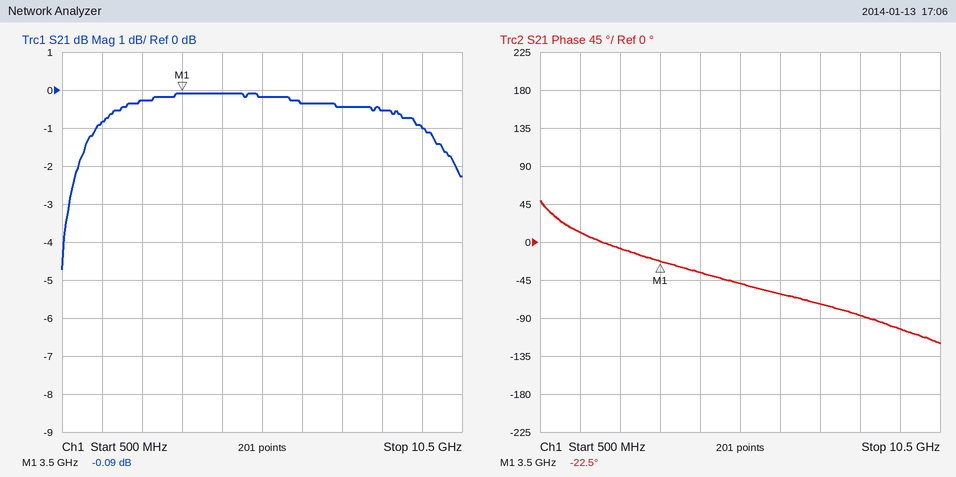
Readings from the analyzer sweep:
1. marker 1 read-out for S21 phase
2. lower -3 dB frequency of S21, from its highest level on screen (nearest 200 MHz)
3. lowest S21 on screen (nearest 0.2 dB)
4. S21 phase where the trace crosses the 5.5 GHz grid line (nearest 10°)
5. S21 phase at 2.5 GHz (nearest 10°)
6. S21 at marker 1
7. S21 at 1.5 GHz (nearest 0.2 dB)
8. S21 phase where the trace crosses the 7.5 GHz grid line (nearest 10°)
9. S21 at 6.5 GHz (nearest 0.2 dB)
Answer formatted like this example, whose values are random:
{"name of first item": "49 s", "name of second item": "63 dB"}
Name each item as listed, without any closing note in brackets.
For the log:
{"marker 1 read-out for S21 phase": "-22.5°", "lower -3 dB frequency of S21, from its highest level on screen": "600 MHz", "lowest S21 on screen": "-4.8 dB", "S21 phase where the trace crosses the 5.5 GHz grid line": "-50°", "S21 phase at 2.5 GHz": "-10°", "S21 at marker 1": "-0.09 dB", "S21 at 1.5 GHz": "-0.8 dB", "S21 phase where the trace crosses the 7.5 GHz grid line": "-70°", "S21 at 6.5 GHz": "-0.4 dB"}
